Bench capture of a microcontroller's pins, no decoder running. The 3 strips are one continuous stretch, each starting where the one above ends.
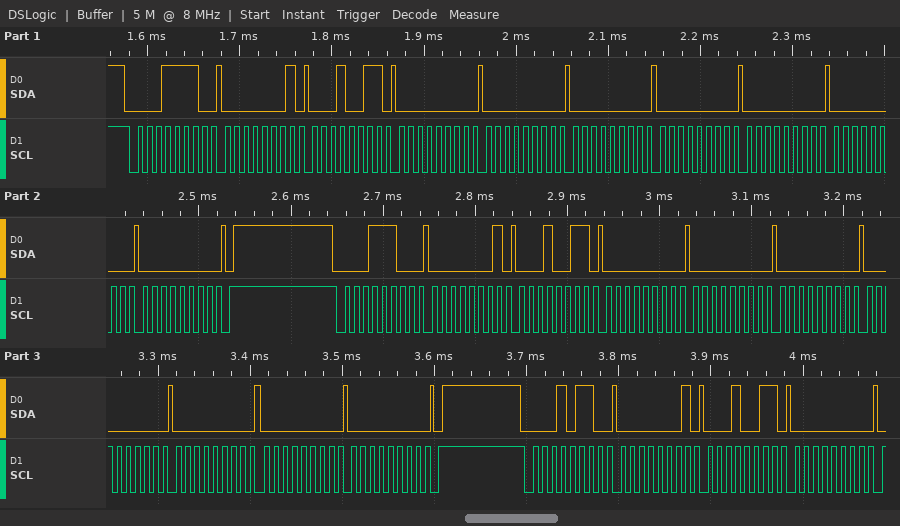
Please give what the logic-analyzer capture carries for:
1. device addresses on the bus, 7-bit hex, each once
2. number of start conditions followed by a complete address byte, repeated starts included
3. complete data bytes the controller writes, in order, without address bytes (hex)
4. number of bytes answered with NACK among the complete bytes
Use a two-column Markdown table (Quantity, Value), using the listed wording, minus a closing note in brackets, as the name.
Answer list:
| Quantity | Value |
|---|---|
| device addresses on the bus, 7-bit hex, each once | 0x0F 0x0E 0x0B |
| number of start conditions followed by a complete address byte, repeated starts included | 3 |
| complete data bytes the controller writes, in order, without address bytes | 01 13 00 00 00 00 00 00 00 01 13 00 00 00 00 00 00 00 01 13 00 |
| number of bytes answered with NACK among the complete bytes | 0 |
